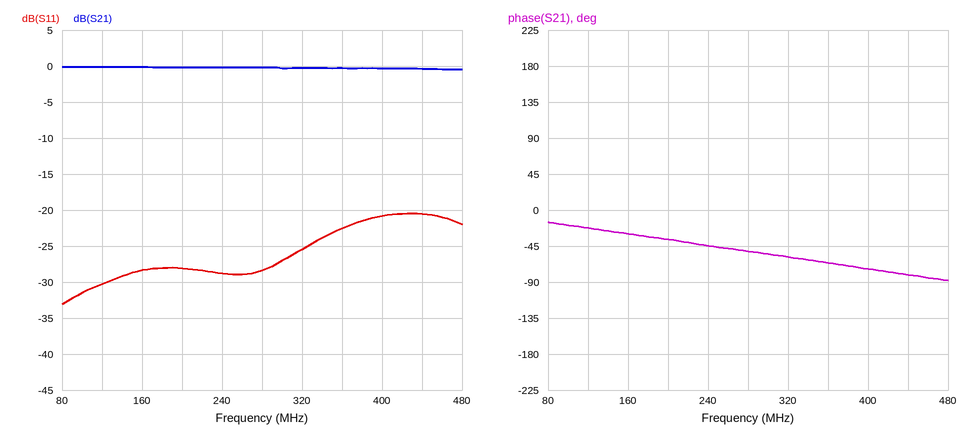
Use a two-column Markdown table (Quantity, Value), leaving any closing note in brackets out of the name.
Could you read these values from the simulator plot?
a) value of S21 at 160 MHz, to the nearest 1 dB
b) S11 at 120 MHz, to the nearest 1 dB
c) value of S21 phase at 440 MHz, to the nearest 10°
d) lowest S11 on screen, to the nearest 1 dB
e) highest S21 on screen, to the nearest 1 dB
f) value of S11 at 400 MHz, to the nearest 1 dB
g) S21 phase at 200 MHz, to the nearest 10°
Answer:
| Quantity | Value |
|---|---|
| value of S21 at 160 MHz, to the nearest 1 dB | 0 dB |
| S11 at 120 MHz, to the nearest 1 dB | -30 dB |
| value of S21 phase at 440 MHz, to the nearest 10° | -80° |
| lowest S11 on screen, to the nearest 1 dB | -33 dB |
| highest S21 on screen, to the nearest 1 dB | 0 dB |
| value of S11 at 400 MHz, to the nearest 1 dB | -21 dB |
| S21 phase at 200 MHz, to the nearest 10° | -40° |
